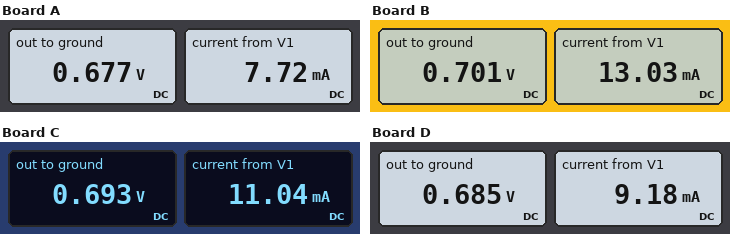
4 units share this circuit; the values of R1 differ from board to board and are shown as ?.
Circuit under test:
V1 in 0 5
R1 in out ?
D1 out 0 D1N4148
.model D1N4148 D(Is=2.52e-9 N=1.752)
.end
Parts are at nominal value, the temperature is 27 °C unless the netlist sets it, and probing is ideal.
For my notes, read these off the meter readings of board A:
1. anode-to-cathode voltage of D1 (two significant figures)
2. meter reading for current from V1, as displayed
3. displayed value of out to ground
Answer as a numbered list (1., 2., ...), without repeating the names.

1. 680 mV
2. 7.72 mA
3. 0.677 V
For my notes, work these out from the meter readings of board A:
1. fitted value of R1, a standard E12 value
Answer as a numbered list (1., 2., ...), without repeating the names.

1. 560 Ω
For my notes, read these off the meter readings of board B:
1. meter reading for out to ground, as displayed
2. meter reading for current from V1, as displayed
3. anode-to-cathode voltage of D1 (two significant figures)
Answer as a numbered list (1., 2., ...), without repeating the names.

1. 0.701 V
2. 13.03 mA
3. 700 mV
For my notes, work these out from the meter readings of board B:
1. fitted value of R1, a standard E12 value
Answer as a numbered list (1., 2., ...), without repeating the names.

1. 330 Ω
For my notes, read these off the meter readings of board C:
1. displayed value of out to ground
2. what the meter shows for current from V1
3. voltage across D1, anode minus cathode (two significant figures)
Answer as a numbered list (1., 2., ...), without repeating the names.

1. 0.693 V
2. 11.04 mA
3. 690 mV
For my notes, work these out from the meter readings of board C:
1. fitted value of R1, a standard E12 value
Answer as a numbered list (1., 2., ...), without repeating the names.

1. 390 Ω
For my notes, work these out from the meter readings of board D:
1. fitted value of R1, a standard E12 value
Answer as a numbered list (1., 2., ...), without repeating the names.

1. 470 Ω
